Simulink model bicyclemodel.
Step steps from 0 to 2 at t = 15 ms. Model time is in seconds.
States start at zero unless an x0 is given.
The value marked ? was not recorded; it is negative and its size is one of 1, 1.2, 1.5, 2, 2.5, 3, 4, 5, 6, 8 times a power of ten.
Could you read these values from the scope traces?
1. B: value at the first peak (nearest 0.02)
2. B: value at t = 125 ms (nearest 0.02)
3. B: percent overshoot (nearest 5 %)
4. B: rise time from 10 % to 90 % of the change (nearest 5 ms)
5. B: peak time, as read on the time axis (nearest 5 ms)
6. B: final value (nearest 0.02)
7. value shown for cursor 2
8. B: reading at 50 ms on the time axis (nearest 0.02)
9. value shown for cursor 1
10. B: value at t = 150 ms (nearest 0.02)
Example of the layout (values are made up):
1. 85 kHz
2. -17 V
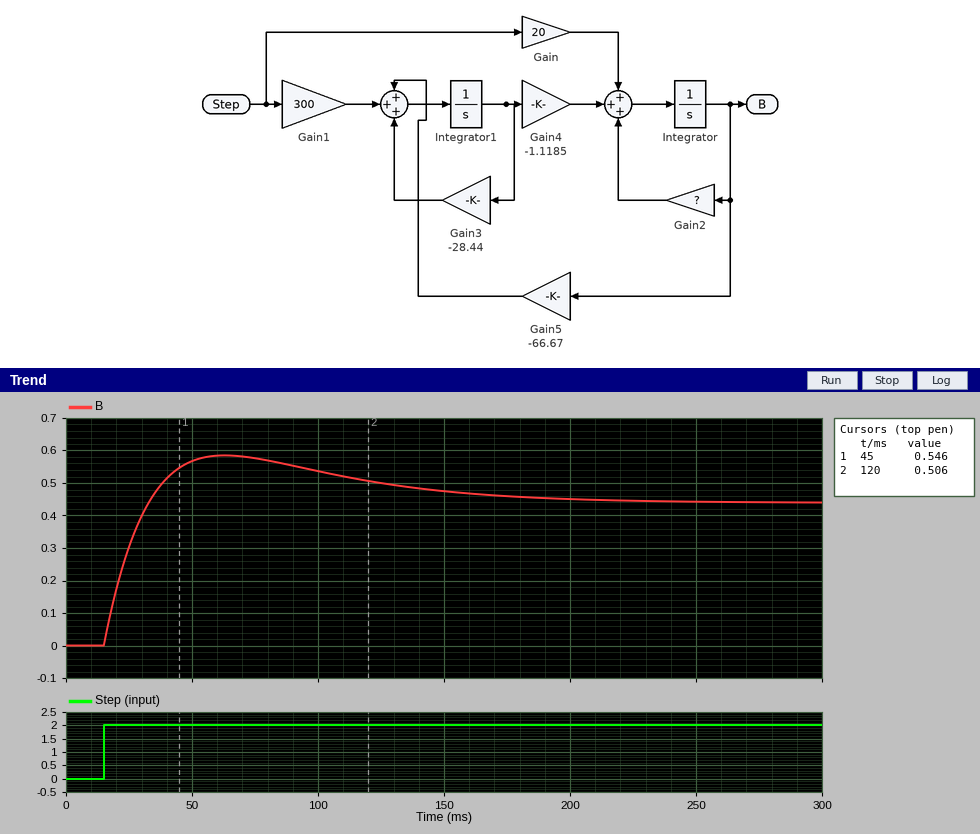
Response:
1. 0.58
2. 0.50
3. 35 %
4. 15 ms
5. 65 ms
6. 0.44
7. 0.506
8. 0.56
9. 0.546
10. 0.48
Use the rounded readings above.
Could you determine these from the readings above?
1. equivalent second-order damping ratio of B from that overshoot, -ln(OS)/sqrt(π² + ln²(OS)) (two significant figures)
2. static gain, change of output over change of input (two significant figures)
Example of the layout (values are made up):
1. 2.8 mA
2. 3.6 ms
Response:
1. 0.32
2. 0.22
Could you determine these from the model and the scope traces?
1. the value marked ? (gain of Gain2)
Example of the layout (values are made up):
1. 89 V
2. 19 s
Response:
1. -40
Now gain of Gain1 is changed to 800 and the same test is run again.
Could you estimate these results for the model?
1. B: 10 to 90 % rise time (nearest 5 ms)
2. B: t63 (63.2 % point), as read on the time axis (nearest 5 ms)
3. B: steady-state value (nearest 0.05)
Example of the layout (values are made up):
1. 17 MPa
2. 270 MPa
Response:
1. 100 ms
2. 125 ms
3. -0.60
